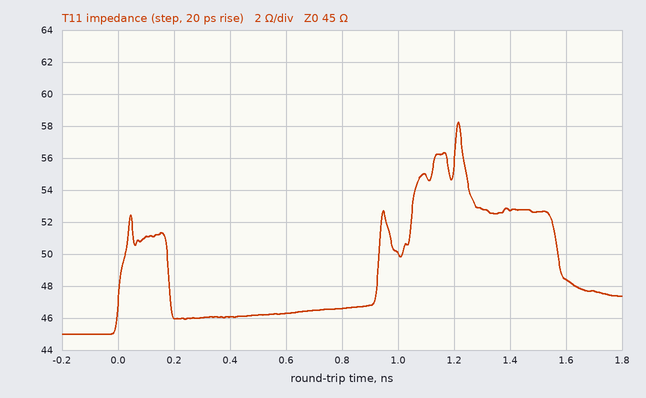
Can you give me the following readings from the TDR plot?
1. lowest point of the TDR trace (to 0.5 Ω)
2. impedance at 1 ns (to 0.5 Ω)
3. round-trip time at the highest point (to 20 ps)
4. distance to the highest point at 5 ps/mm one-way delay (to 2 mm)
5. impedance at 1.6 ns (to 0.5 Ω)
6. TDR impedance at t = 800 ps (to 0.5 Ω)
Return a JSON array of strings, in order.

["45.0 Ω", "50.0 Ω", "1.22 ns", "122 mm", "48.5 Ω", "46.5 Ω"]
